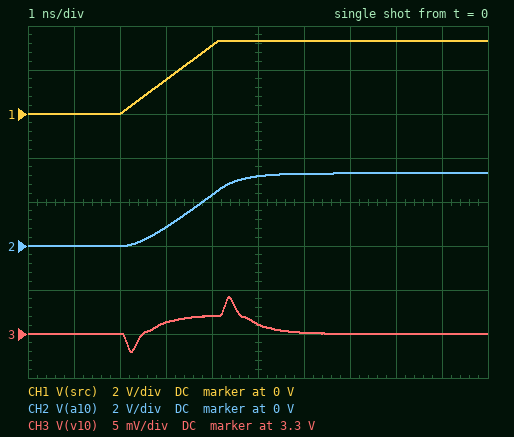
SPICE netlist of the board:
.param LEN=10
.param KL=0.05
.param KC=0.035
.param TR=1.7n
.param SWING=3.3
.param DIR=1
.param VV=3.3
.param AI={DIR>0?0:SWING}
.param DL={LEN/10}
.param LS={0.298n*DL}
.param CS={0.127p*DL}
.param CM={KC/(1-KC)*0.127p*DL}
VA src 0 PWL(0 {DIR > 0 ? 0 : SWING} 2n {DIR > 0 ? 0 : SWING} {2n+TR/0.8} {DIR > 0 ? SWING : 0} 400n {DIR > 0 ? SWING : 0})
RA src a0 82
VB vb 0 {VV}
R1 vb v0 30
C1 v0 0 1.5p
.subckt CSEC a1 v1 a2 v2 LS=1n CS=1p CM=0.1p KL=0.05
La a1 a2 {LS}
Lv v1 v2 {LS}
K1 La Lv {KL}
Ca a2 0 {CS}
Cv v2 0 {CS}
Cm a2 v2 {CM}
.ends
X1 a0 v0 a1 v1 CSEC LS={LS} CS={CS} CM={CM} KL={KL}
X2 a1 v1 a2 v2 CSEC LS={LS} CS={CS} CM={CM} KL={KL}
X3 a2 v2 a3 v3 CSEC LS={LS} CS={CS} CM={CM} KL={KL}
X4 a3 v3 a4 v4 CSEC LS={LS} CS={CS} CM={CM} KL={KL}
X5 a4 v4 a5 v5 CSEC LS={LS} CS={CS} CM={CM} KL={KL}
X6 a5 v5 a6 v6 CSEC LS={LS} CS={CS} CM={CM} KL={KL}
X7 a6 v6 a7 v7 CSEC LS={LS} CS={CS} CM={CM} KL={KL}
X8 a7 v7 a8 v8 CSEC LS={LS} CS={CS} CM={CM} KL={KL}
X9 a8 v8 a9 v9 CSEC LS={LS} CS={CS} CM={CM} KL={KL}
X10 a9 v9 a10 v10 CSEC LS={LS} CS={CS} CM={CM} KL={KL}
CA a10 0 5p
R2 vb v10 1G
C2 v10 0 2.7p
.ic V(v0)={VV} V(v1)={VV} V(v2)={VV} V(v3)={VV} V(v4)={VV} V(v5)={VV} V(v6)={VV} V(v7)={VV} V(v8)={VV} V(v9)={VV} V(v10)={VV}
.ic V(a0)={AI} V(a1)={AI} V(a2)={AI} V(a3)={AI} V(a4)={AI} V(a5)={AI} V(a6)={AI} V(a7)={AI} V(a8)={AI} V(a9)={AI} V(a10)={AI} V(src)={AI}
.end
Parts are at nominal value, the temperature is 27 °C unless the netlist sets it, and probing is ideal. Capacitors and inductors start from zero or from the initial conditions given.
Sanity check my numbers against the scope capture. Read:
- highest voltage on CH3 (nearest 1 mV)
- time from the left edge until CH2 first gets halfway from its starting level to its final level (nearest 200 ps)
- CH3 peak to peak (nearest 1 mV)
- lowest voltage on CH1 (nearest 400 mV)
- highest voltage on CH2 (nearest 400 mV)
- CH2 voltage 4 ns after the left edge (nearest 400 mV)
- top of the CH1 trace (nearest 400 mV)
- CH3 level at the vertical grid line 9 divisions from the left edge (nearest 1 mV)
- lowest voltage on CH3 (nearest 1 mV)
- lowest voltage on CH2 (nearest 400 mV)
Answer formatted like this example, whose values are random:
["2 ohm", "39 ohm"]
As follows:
["3.304 V", "3.6 ns", "6 mV", "0 V", "3.2 V", "2.4 V", "3.2 V", "3.300 V", "3.298 V", "0 V"]
